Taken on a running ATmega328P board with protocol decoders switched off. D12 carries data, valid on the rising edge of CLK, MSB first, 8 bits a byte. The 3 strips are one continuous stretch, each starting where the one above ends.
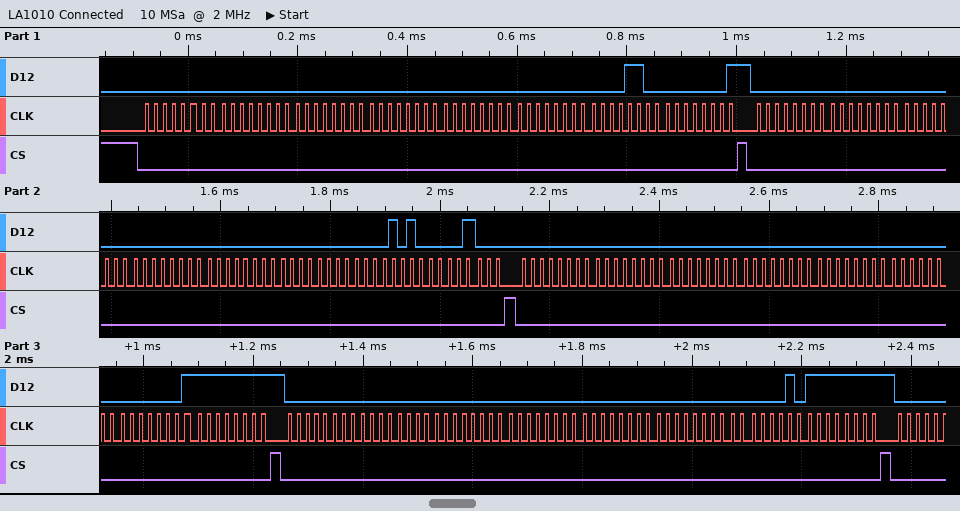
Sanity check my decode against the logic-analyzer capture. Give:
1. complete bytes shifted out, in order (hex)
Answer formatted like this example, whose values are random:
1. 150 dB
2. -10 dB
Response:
1. 0x00 0x00 0x00 0x00 0x00 0x00 0x0C 0x01 0x00 0x00 0x00 0x00 0x00 0x00 0x0A 0x08 0x00 0x00 0x00 0x00 0x00 0x00 0x01 0xFF 0x00 0x00 0x00 0x00 0x00 0x00 0x02 0xFF
